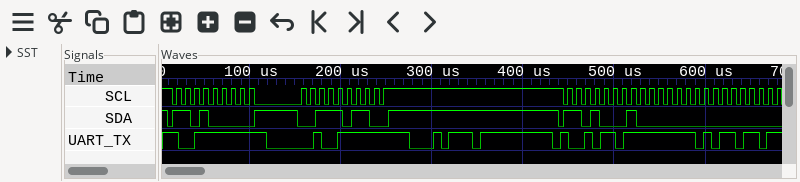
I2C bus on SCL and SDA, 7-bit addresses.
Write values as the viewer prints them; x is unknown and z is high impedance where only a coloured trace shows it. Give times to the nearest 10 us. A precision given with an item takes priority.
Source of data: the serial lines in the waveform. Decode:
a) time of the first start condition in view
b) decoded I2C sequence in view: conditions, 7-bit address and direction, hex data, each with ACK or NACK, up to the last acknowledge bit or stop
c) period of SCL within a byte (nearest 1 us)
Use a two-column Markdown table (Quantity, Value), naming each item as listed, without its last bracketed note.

| Quantity | Value |
|---|---|
| time of the first start condition in view | 10 us |
| decoded I2C sequence in view: conditions, 7-bit address and direction, hex data, each with ACK or NACK, up to the last acknowledge bit or stop | start, address 68 write ACK, 3B ACK, stop, start, address 68 read ACK, 00 ACK |
| period of SCL within a byte | 10 us |
